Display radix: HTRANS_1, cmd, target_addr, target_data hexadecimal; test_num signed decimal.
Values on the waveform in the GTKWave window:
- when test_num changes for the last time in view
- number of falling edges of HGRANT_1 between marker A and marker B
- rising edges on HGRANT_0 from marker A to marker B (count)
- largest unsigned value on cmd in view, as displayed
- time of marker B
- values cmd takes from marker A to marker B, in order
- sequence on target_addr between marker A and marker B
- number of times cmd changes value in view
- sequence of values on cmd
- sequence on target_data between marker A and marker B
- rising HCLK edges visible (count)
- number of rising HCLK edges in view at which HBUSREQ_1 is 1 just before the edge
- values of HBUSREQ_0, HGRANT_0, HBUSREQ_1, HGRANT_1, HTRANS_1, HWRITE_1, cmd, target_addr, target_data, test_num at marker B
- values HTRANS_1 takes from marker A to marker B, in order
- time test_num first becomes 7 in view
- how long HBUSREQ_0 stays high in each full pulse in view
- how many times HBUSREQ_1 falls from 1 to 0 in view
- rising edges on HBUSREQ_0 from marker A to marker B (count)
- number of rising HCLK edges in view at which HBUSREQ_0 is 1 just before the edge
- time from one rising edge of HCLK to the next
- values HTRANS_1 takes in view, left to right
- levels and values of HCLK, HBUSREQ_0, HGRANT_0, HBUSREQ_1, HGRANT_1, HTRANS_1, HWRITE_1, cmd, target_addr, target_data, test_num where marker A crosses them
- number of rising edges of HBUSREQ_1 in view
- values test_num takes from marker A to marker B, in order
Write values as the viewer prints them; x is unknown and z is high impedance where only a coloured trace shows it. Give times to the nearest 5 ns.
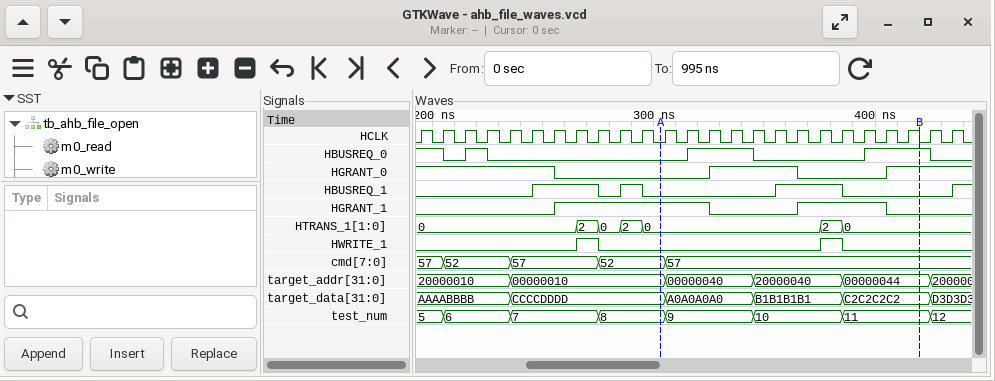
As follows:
425 ns
2
2
57
420 ns
52, 57
00000010, 00000040, 20000040, 00000044
4
57, 52, 57, 52, 57
CCCCDDDD, A0A0A0A0, B1B1B1B1, C2C2C2C2
25
7
HBUSREQ_0=1, HGRANT_0=1, HBUSREQ_1=0, HGRANT_1=0, HTRANS_1=0, HWRITE_1=0, cmd=57, target_addr=00000044, target_data=C2C2C2C2, test_num=11
0, 2, 0
235 ns
10 ns, 30 ns, 30 ns
3
2
9
10 ns
0, 2, 0, 2, 0, 2, 0
HCLK=0, HBUSREQ_0=0, HGRANT_0=0, HBUSREQ_1=0, HGRANT_1=1, HTRANS_1=0, HWRITE_1=0, cmd=52, target_addr=00000010, target_data=CCCCDDDD, test_num=8
4
8, 9, 10, 11
